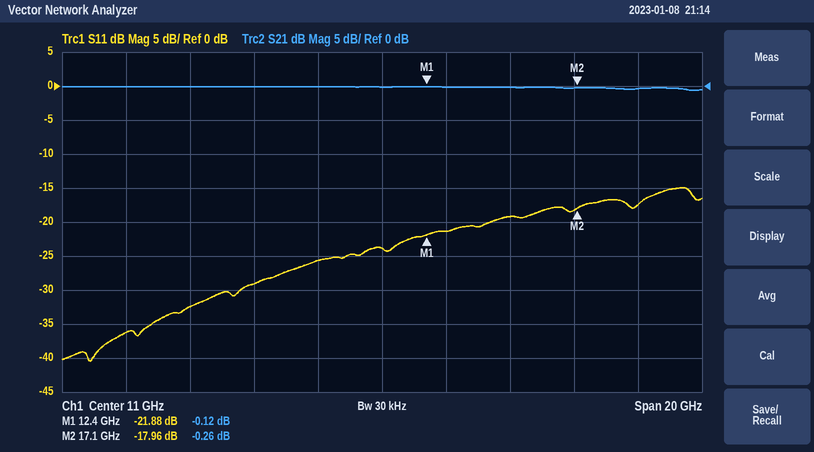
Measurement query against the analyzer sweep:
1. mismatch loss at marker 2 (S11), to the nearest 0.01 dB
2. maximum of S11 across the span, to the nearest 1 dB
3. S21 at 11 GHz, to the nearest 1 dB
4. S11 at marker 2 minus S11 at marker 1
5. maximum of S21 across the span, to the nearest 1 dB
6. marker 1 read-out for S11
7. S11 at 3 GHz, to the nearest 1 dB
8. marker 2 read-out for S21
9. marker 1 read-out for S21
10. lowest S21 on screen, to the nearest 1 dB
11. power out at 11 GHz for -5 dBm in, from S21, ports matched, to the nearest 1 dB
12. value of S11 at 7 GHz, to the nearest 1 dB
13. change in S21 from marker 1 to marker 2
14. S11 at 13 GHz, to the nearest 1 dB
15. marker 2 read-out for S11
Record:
0.07 dB
-15 dB
0 dB
3.92 dB
0 dB
-21.88 dB
-36 dB
-0.26 dB
-0.12 dB
-1 dB
-5 dBm
-29 dB
-0.14 dB
-21 dB
-17.96 dB
